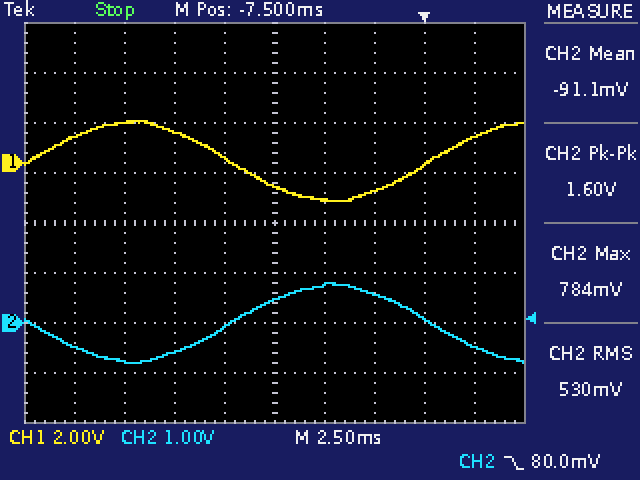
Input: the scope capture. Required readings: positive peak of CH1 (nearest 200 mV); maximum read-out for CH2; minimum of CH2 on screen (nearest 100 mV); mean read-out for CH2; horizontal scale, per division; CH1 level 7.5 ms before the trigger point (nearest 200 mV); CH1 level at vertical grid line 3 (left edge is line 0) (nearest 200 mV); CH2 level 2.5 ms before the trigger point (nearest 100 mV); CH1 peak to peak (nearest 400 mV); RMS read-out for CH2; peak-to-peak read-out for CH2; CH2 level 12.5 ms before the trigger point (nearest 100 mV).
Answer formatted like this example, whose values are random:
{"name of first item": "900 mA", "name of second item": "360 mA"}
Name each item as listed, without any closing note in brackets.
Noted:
{"positive peak of CH1": "1.6 V", "maximum read-out for CH2": "784 mV", "minimum of CH2 on screen": "-800 mV", "mean read-out for CH2": "-91.1 mV", "horizontal scale, per division": "2.5 ms", "CH1 level 7.5 ms before the trigger point": "-1.0 V", "CH1 level at vertical grid line 3 (left edge is line 0)": "1.2 V", "CH2 level 2.5 ms before the trigger point": "600 mV", "CH1 peak to peak": "3.2 V", "RMS read-out for CH2": "530 mV", "peak-to-peak read-out for CH2": "1.60 V", "CH2 level 12.5 ms before the trigger point": "-600 mV"}
